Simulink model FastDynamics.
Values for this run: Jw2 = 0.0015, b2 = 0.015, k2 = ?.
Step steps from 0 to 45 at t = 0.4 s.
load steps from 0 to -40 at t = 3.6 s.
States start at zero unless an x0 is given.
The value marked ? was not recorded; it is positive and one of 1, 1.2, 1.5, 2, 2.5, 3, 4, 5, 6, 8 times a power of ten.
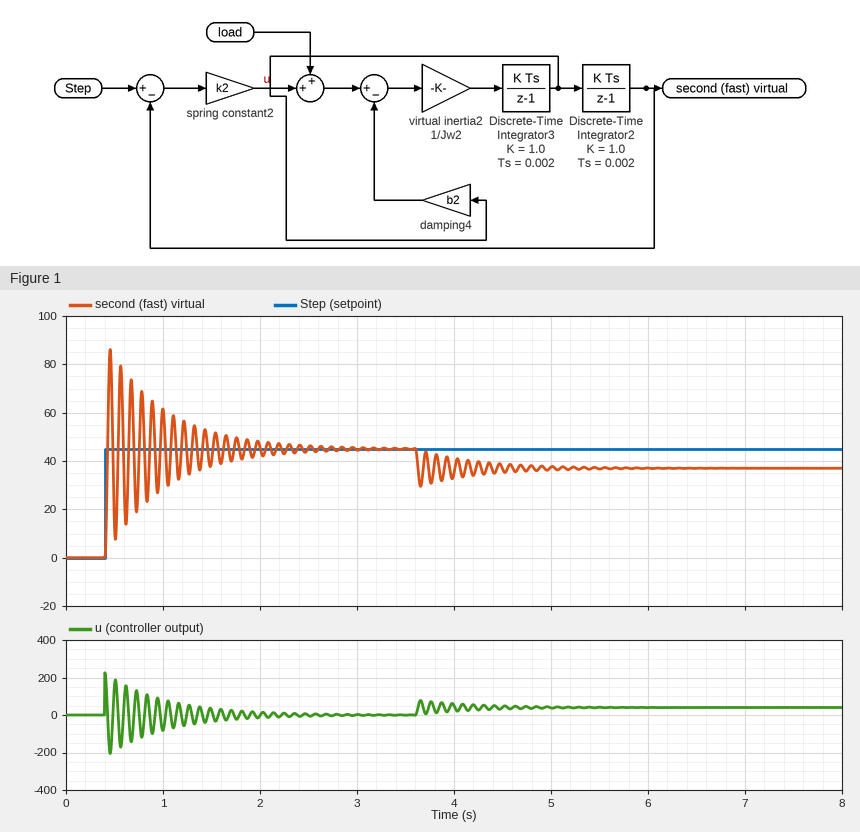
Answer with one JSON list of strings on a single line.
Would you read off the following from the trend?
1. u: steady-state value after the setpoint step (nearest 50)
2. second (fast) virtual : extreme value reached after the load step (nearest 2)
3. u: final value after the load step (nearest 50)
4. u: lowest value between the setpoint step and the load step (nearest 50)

["0", "30", "50", "-200"]
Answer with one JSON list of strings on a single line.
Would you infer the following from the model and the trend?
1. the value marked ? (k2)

["5"]
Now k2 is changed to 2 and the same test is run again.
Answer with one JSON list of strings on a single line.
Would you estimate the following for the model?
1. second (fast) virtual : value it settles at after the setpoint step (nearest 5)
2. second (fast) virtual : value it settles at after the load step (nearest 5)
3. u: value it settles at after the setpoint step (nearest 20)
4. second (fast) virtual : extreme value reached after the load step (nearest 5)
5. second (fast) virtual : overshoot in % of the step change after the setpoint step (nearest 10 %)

["45", "25", "0", "10", "70 %"]
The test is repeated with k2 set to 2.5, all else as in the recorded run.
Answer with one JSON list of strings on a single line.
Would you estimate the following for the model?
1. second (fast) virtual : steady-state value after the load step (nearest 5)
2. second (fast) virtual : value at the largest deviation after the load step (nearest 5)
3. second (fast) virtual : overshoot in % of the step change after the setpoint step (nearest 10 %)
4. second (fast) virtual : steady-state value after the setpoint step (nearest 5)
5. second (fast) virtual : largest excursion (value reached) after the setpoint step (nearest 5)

["30", "15", "80 %", "45", "80"]
